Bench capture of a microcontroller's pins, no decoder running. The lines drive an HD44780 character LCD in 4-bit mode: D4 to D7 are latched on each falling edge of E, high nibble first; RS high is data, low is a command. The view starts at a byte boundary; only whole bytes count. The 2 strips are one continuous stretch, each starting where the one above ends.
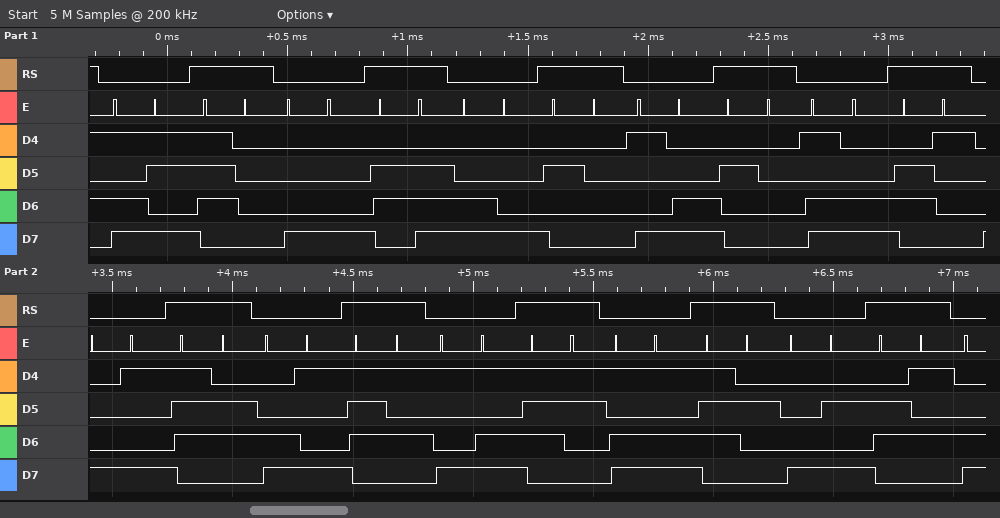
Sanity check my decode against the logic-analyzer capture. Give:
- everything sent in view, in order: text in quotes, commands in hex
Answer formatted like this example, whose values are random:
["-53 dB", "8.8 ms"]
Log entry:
["0xDB \"p\" 0x88 \"n\" 0xC8 \" \" 0x9C \" \" 0xDC \"a\" 0x89 \"v\" 0xC9 \"u\" 0x9D \"s\" 0xDD \"r\" 0x8A \"e\""]
